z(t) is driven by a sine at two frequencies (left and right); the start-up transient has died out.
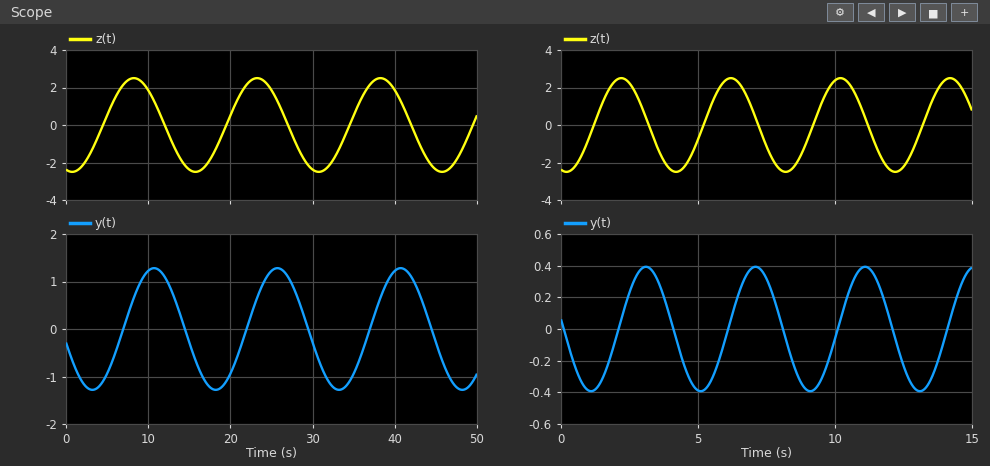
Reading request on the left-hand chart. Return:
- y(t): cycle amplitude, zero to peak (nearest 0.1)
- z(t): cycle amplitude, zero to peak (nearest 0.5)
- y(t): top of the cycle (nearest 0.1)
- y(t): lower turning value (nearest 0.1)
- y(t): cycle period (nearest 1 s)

1.3
2.5
1.3
-1.3
15 s
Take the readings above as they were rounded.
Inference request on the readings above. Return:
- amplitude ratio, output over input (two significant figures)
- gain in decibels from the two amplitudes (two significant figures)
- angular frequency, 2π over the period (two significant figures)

0.52
-5.7 dB
0.42 rad/s
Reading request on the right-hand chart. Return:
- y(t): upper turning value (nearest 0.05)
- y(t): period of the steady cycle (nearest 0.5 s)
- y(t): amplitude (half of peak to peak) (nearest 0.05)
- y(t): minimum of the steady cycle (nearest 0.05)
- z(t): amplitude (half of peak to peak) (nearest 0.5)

0.40
4.0 s
0.40
-0.40
2.5
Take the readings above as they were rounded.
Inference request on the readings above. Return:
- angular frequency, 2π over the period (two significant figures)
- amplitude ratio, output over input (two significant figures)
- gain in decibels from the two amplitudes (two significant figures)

1.6 rad/s
0.16
-16 dB
